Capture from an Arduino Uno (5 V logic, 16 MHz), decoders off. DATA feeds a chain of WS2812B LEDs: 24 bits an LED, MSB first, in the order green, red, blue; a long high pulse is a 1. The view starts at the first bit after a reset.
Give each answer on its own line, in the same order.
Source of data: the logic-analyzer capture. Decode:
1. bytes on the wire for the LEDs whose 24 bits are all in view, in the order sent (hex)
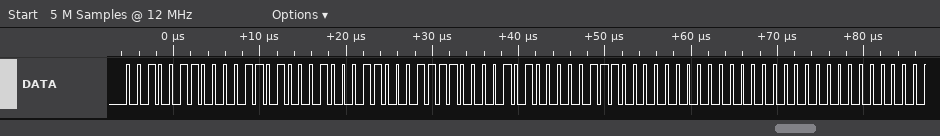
26 1A 23 1E 14 1C 00 00 00
